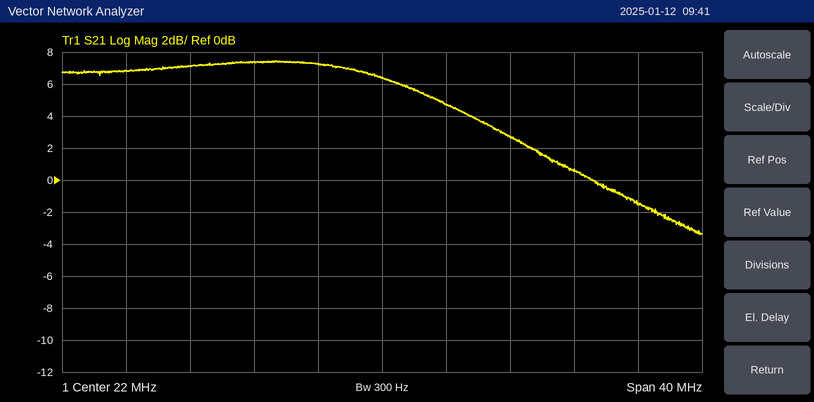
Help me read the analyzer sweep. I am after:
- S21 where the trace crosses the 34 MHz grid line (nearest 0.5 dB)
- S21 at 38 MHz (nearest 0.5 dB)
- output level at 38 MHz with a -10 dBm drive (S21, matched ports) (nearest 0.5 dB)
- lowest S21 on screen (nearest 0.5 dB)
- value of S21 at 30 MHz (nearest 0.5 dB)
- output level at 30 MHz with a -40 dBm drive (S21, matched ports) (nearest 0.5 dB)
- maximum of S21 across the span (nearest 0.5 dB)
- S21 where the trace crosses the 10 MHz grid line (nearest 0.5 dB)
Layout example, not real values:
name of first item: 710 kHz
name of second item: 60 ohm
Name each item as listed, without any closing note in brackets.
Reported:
S21 where the trace crosses the 34 MHz grid line: 0.5 dB
S21 at 38 MHz: -1.5 dB
output level at 38 MHz with a -10 dBm drive (S21, matched ports): -11.5 dBm
lowest S21 on screen: -3.5 dB
value of S21 at 30 MHz: 2.5 dB
output level at 30 MHz with a -40 dBm drive (S21, matched ports): -37.5 dBm
maximum of S21 across the span: 7.5 dB
S21 where the trace crosses the 10 MHz grid line: 7.0 dB
